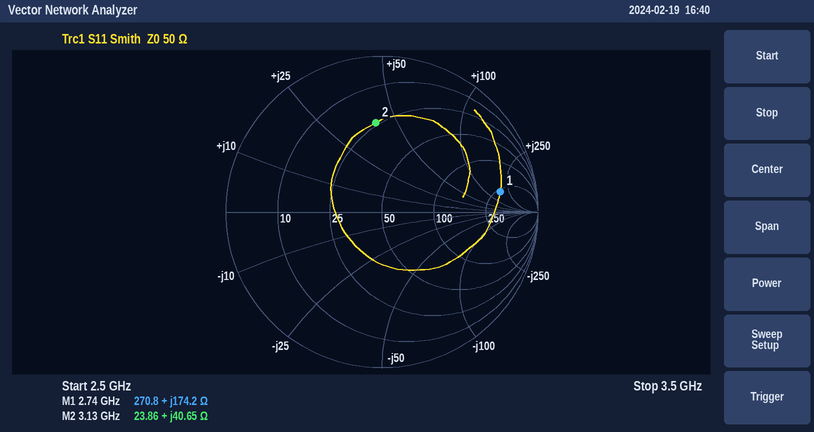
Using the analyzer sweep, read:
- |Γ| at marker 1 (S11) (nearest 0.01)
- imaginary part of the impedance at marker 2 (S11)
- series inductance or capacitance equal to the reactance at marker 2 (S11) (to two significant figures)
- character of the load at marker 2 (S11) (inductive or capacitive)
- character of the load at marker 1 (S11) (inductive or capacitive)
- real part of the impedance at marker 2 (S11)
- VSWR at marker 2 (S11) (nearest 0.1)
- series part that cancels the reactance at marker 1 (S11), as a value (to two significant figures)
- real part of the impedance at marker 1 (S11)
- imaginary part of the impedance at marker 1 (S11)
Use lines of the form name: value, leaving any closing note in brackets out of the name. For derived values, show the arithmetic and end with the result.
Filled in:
|Γ| at marker 1 (S11): 0.77
imaginary part of the impedance at marker 2: +40.65 Ω
series inductance or capacitance equal to the reactance at marker 2 (S11): L = 40.65 Ω/(2π × 3.13 GHz) ≈ 2.1 nH
character of the load at marker 2 (S11): inductive
character of the load at marker 1 (S11): inductive
real part of the impedance at marker 2: 23.86 Ω
VSWR at marker 2 (S11): 3.7
series part that cancels the reactance at marker 1 (S11), as a value: C = 1/(2π × 2.74 GHz × 174.2 Ω) ≈ 333 fF, so 330 fF to two significant figures
real part of the impedance at marker 1: 270.8 Ω
imaginary part of the impedance at marker 1: +174.2 Ω
